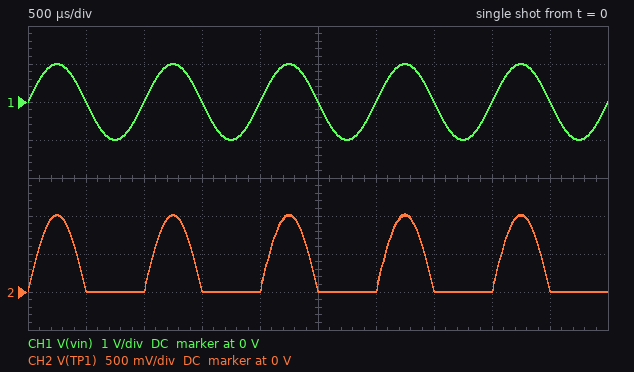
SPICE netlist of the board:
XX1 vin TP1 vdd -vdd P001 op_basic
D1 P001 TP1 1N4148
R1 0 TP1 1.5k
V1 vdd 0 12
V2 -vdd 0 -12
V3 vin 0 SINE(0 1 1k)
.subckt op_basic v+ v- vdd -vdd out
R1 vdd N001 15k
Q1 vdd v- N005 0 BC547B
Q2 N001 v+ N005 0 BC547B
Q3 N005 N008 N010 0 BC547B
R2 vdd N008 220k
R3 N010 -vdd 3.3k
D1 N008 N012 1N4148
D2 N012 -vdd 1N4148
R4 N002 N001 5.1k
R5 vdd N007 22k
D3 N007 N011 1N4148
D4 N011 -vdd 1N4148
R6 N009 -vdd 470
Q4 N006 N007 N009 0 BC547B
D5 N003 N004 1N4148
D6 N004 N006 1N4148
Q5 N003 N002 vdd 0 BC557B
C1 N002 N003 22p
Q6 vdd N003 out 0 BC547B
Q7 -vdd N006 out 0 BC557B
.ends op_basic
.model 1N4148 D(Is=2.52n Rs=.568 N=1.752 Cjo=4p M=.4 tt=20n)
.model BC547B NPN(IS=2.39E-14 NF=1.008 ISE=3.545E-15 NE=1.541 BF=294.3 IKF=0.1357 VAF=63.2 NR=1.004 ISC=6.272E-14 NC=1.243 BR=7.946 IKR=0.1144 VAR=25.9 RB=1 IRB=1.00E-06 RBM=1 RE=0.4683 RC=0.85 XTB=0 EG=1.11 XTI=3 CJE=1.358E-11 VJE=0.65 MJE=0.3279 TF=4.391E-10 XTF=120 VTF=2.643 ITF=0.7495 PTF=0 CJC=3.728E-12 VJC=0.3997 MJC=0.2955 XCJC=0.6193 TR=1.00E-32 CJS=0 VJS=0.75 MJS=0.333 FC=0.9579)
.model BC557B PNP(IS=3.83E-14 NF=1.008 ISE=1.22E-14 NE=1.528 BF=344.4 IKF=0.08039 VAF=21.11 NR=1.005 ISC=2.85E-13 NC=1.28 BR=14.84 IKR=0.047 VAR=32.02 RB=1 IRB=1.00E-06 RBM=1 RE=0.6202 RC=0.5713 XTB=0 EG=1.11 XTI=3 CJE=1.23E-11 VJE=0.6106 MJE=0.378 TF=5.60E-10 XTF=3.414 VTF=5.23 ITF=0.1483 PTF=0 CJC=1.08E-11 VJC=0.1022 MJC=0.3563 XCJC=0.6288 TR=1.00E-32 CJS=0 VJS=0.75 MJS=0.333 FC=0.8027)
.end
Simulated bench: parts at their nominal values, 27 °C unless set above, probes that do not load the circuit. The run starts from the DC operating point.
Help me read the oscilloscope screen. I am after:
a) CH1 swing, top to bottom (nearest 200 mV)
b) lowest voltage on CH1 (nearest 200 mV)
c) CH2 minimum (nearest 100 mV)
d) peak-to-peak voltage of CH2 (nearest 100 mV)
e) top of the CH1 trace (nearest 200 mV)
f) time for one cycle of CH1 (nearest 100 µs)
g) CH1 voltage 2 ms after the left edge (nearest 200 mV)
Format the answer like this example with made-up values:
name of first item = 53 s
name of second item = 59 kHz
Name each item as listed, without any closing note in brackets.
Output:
CH1 swing, top to bottom = 2.0 V
lowest voltage on CH1 = -1.0 V
CH2 minimum = 0 V
peak-to-peak voltage of CH2 = 1.0 V
top of the CH1 trace = 1.0 V
time for one cycle of CH1 = 1.0 ms
CH1 voltage 2 ms after the left edge = 0 V
